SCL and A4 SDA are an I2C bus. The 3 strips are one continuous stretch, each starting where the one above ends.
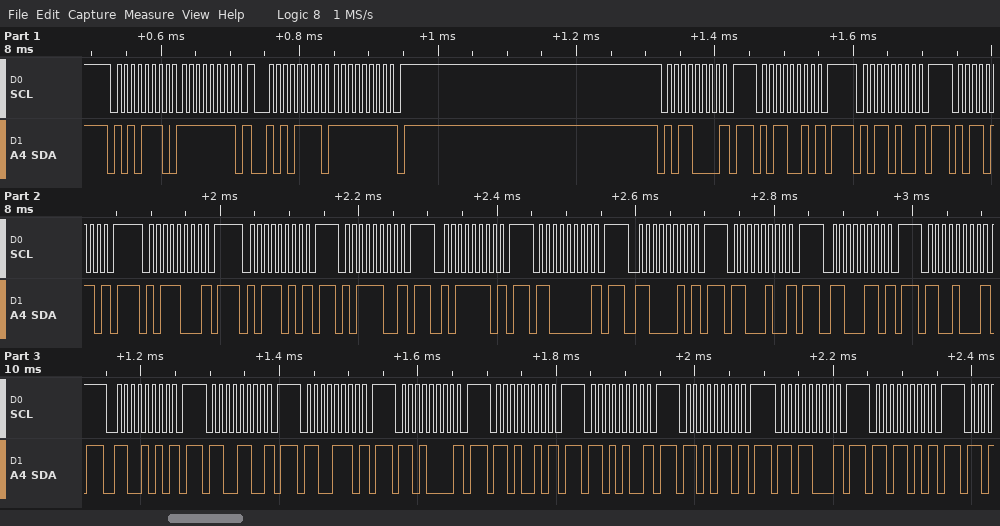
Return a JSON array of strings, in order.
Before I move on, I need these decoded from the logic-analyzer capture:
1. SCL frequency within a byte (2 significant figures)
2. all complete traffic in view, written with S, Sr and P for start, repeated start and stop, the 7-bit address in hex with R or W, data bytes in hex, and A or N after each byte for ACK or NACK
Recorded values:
["100 kHz", "S 57W A FF A Sr 57R A FF N P S 58W N P S 59W N P S 5AW N P S 5BW N P S 5CW N P S 5DW N P S 5EW N P S 5FW N P S 60W N P S 61W N P S 62W N P S 63W N P S 64W N P S 65W N P S 66W N P S 67W N P S 68W N P S 69W N P S 6AW N P S 6BW N P S 6CW N P S 6DW N P"]
